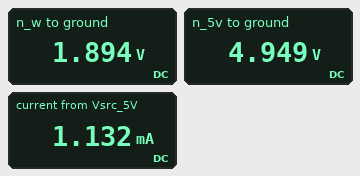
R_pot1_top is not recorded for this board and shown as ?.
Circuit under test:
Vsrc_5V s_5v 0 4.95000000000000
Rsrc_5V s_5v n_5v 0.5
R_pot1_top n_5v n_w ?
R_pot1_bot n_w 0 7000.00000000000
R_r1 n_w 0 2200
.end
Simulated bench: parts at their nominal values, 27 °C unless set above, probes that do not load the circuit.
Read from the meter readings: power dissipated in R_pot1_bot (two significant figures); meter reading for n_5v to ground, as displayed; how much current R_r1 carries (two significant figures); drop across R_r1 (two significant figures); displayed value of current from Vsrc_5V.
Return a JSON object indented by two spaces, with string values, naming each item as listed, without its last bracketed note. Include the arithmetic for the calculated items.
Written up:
{
  "power dissipated in R_pot1_bot": "(1.894 V)^2 / 7 kΩ = 510 µW",
  "meter reading for n_5v to ground, as displayed": "4.949 V",
  "how much current R_r1 carries": "(1.894 V) / 2.2 kΩ = 860 µA",
  "drop across R_r1": "1.894 V = 1.9 V",
  "displayed value of current from Vsrc_5V": "1.132 mA"
}
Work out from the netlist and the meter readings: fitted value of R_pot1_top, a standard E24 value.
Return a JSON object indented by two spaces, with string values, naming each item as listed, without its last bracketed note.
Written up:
{
  "fitted value of R_pot1_top, a standard E24 value": "2.7 kΩ"
}
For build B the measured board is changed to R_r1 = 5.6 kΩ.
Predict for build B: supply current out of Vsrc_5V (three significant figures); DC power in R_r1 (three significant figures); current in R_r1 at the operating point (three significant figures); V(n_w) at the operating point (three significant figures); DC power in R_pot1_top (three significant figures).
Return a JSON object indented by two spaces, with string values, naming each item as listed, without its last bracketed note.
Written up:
{
  "supply current out of Vsrc_5V": "852 µA",
  "DC power in R_r1": "1.25 mW",
  "current in R_r1 at the operating point": "473 µA",
  "V(n_w) at the operating point": "2.65 V",
  "DC power in R_pot1_top": "1.96 mW"
}
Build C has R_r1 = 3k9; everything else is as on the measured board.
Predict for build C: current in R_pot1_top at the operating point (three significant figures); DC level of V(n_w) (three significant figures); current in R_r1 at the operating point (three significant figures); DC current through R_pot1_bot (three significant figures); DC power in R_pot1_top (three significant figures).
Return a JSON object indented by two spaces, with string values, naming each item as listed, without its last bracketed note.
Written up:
{
  "current in R_pot1_top at the operating point": "951 µA",
  "DC level of V(n_w)": "2.38 V",
  "current in R_r1 at the operating point": "611 µA",
  "DC current through R_pot1_bot": "340 µA",
  "DC power in R_pot1_top": "2.44 mW"
}
